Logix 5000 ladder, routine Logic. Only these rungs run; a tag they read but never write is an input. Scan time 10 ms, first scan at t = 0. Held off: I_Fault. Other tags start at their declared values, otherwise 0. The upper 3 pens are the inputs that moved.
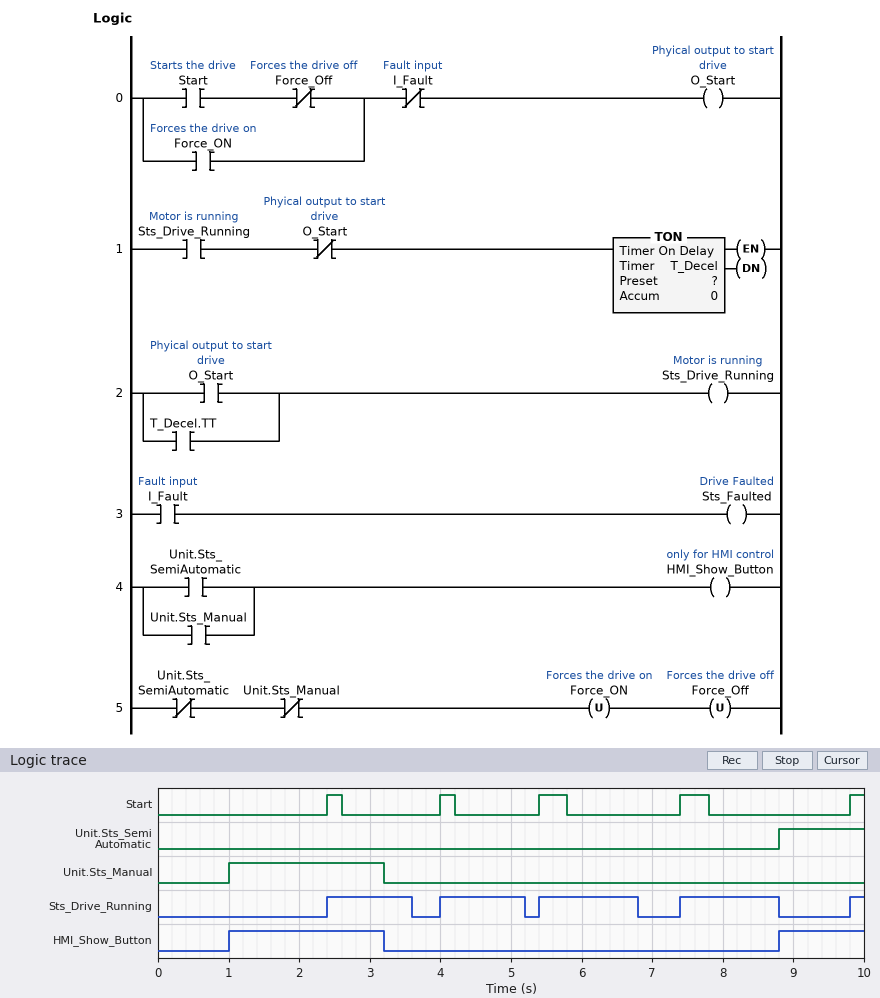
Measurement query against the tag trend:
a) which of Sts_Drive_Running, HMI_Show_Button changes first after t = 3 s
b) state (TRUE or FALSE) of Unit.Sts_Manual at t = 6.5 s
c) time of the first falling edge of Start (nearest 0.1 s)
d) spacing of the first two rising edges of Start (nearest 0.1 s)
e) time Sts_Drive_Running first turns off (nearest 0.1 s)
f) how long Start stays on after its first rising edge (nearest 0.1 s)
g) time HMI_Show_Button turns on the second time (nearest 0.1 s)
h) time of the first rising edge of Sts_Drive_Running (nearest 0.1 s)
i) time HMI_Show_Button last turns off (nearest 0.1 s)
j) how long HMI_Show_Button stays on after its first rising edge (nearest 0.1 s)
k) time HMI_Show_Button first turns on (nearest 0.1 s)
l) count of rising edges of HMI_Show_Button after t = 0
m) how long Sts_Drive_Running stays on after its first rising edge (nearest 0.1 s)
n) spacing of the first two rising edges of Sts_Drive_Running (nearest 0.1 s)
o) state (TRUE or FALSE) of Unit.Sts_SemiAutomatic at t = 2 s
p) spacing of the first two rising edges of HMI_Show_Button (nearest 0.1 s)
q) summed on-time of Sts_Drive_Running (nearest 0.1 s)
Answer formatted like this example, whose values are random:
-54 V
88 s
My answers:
HMI_Show_Button
FALSE
2.6 s
1.6 s
3.6 s
0.2 s
8.8 s
2.4 s
3.2 s
2.2 s
1.0 s
2
1.2 s
1.6 s
FALSE
7.8 s
5.4 s
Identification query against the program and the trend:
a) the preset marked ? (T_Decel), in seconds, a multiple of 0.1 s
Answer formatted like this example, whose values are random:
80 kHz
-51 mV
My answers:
1.0 s
